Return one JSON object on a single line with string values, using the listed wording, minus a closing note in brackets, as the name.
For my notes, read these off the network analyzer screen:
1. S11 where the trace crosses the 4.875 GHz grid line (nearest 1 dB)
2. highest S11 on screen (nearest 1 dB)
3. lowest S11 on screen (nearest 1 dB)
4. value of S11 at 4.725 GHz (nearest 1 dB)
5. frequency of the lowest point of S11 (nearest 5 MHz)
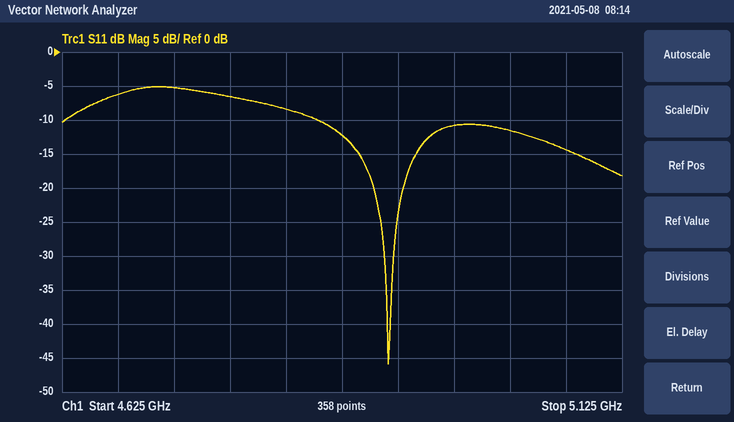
{"S11 where the trace crosses the 4.875 GHz grid line": "-12 dB", "highest S11 on screen": "-5 dB", "lowest S11 on screen": "-46 dB", "value of S11 at 4.725 GHz": "-5 dB", "frequency of the lowest point of S11": "4.915 GHz"}
